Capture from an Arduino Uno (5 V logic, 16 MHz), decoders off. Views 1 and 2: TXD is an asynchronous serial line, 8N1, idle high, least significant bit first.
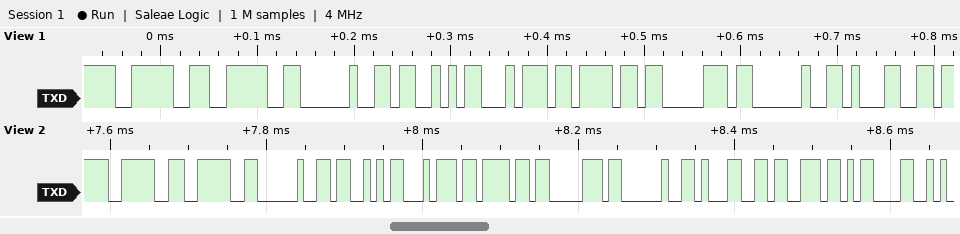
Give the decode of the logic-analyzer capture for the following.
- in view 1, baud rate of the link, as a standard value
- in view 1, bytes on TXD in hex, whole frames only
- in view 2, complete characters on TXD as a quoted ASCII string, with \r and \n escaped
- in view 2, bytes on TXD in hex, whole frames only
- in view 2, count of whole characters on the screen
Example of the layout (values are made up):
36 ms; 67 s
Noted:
115200 baud; 3E 3E 20 53 74 6F 70 20 31; ">> Stop 1s\r"; 3E 3E 20 53 74 6F 70 20 31 73 0D; 11
